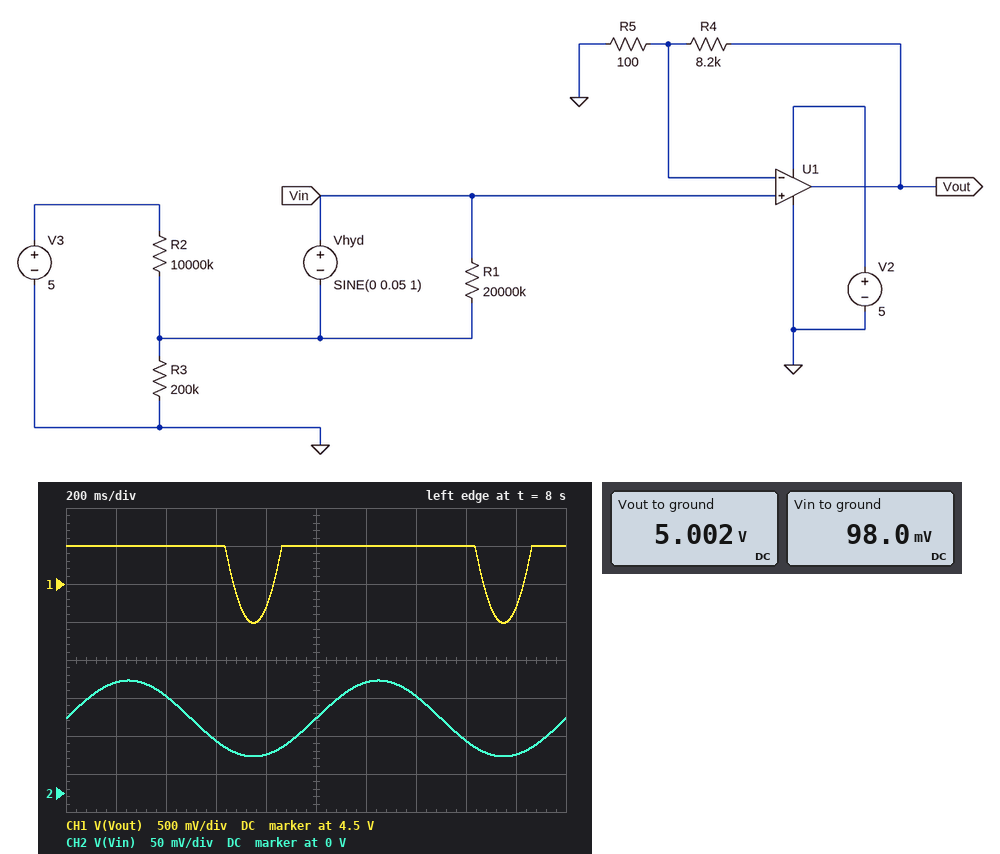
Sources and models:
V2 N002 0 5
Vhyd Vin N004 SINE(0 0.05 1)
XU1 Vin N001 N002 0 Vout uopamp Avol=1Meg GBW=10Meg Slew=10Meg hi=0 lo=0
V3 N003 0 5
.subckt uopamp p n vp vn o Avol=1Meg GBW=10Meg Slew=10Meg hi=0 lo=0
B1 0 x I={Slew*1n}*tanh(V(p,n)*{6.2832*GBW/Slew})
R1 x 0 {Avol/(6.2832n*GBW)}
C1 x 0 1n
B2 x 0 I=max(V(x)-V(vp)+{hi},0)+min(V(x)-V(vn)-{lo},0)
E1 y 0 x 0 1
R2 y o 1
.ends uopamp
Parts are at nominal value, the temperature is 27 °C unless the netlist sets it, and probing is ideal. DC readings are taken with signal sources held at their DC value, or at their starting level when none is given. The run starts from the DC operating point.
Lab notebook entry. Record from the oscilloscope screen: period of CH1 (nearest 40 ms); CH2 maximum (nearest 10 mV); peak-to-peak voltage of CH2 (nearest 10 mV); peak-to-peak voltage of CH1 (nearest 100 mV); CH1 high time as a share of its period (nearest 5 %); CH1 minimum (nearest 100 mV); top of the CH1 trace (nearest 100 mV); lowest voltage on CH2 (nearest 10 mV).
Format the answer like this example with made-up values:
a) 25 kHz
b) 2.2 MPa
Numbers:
a) 1.00 s
b) 150 mV
c) 100 mV
d) 1.0 V
e) 85 %
f) 4.0 V
g) 5.0 V
h) 50 mV
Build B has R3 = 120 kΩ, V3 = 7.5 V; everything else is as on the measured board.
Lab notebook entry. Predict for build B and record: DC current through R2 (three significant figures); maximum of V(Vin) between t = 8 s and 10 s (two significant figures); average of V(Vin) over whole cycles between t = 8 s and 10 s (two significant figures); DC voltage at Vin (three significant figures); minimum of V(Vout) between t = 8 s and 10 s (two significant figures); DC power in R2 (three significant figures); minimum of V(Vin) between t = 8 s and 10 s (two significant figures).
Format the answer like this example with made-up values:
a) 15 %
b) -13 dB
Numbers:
a) 741 nA
b) 140 mV
c) 89 mV
d) 88.9 mV
e) 3.2 V
f) 5.49 µW
g) 39 mV
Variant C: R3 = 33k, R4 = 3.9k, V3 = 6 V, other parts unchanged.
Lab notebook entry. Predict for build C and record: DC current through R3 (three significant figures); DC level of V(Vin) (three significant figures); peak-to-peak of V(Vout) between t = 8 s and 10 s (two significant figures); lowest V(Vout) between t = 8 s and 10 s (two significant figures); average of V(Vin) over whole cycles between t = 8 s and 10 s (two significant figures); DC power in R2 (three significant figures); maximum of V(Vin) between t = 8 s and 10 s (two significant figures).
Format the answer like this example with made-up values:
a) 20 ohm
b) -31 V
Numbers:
a) 598 nA
b) 19.7 mV
c) 2.8 V
d) -1.9 mV
e) 20 mV
f) 3.58 µW
g) 70 mV
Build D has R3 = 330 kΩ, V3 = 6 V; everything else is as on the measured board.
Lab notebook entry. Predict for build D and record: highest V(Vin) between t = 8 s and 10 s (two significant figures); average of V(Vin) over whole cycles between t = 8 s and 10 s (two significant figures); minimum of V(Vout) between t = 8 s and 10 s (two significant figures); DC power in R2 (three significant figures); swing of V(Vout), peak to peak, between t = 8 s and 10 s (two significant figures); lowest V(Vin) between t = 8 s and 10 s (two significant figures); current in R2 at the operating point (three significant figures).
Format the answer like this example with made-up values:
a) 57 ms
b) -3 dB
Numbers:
a) 240 mV
b) 190 mV
c) 5.0 V
d) 3.37 µW
e) 3.4 mV
f) 140 mV
g) 581 nA
